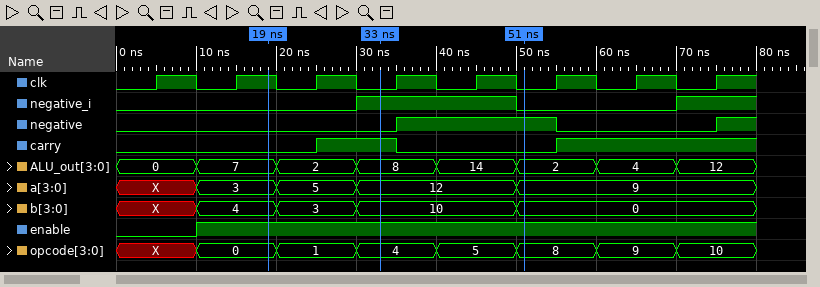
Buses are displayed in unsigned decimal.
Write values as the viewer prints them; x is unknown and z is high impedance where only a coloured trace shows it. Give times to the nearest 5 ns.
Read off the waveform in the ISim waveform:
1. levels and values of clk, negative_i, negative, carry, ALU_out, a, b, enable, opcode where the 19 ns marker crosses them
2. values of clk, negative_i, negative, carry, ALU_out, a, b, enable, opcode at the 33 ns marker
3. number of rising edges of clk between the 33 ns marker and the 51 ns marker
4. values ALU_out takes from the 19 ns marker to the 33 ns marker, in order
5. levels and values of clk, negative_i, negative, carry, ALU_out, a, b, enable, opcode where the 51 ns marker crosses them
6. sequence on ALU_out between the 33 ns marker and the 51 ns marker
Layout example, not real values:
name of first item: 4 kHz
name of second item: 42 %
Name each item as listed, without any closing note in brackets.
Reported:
levels and values of clk, negative_i, negative, carry, ALU_out, a, b, enable, opcode where the 19 ns marker crosses them: clk=1, negative_i=0, negative=0, carry=0, ALU_out=7, a=3, b=4, enable=1, opcode=0
values of clk, negative_i, negative, carry, ALU_out, a, b, enable, opcode at the 33 ns marker: clk=0, negative_i=1, negative=0, carry=1, ALU_out=8, a=12, b=10, enable=1, opcode=4
number of rising edges of clk between the 33 ns marker and the 51 ns marker: 2
values ALU_out takes from the 19 ns marker to the 33 ns marker, in order: 7, 2, 8
levels and values of clk, negative_i, negative, carry, ALU_out, a, b, enable, opcode where the 51 ns marker crosses them: clk=0, negative_i=0, negative=1, carry=0, ALU_out=2, a=9, b=0, enable=1, opcode=8
sequence on ALU_out between the 33 ns marker and the 51 ns marker: 8, 14, 2
